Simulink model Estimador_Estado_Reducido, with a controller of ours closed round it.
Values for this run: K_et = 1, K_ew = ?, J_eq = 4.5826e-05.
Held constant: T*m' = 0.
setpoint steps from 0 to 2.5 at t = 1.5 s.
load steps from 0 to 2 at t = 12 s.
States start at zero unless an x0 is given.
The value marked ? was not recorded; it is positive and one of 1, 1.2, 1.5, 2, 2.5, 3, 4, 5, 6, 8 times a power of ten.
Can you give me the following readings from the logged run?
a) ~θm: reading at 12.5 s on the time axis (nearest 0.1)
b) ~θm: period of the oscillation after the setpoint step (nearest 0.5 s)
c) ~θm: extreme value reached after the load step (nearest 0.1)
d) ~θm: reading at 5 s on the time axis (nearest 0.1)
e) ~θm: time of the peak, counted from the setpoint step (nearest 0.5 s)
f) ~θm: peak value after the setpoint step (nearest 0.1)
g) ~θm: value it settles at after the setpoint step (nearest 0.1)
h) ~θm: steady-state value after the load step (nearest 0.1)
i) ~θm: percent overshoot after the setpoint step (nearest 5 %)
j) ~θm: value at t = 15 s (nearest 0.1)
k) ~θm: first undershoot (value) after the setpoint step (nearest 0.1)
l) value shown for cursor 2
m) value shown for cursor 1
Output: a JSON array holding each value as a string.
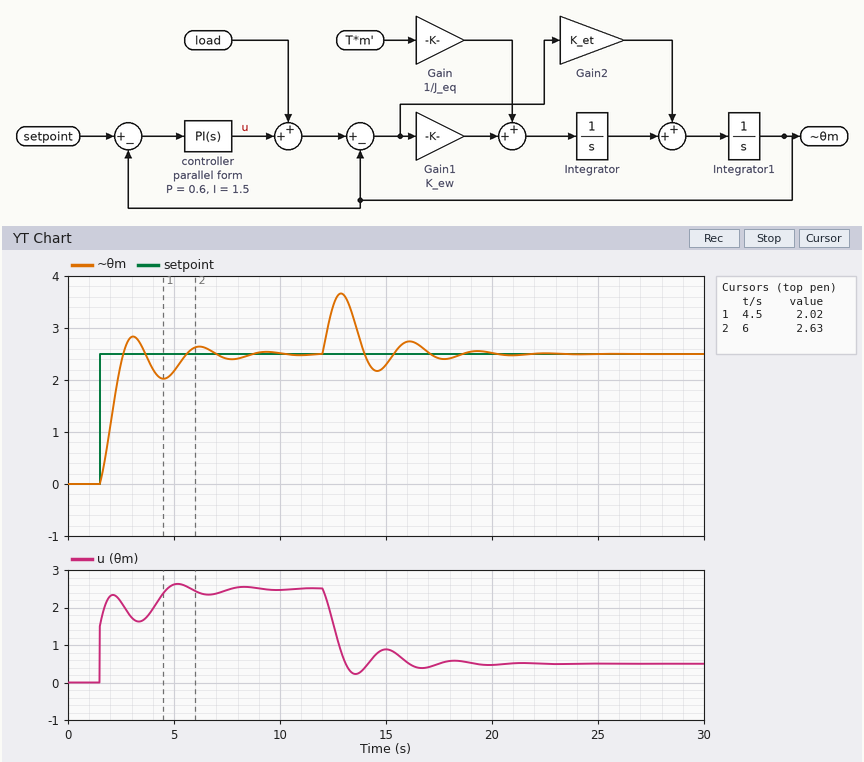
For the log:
["3.4", "3.0 s", "3.7", "2.2", "1.5 s", "2.8", "2.5", "2.5", "15 %", "2.3", "2.0", "2.63", "2.02"]
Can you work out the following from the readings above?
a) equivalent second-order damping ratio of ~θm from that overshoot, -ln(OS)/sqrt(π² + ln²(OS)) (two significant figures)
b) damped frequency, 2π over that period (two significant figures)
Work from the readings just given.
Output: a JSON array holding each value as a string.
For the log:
["0.52", "2.1 rad/s"]
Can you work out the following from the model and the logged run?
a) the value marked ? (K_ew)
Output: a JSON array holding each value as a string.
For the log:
["2"]
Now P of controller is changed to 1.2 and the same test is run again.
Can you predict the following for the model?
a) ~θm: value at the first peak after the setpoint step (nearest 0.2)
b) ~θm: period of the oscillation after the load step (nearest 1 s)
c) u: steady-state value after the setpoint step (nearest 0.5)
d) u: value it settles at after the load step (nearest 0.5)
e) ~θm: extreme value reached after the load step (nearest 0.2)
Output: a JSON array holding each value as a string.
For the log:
["2.6", "3 s", "2.5", "0.5", "3.4"]
